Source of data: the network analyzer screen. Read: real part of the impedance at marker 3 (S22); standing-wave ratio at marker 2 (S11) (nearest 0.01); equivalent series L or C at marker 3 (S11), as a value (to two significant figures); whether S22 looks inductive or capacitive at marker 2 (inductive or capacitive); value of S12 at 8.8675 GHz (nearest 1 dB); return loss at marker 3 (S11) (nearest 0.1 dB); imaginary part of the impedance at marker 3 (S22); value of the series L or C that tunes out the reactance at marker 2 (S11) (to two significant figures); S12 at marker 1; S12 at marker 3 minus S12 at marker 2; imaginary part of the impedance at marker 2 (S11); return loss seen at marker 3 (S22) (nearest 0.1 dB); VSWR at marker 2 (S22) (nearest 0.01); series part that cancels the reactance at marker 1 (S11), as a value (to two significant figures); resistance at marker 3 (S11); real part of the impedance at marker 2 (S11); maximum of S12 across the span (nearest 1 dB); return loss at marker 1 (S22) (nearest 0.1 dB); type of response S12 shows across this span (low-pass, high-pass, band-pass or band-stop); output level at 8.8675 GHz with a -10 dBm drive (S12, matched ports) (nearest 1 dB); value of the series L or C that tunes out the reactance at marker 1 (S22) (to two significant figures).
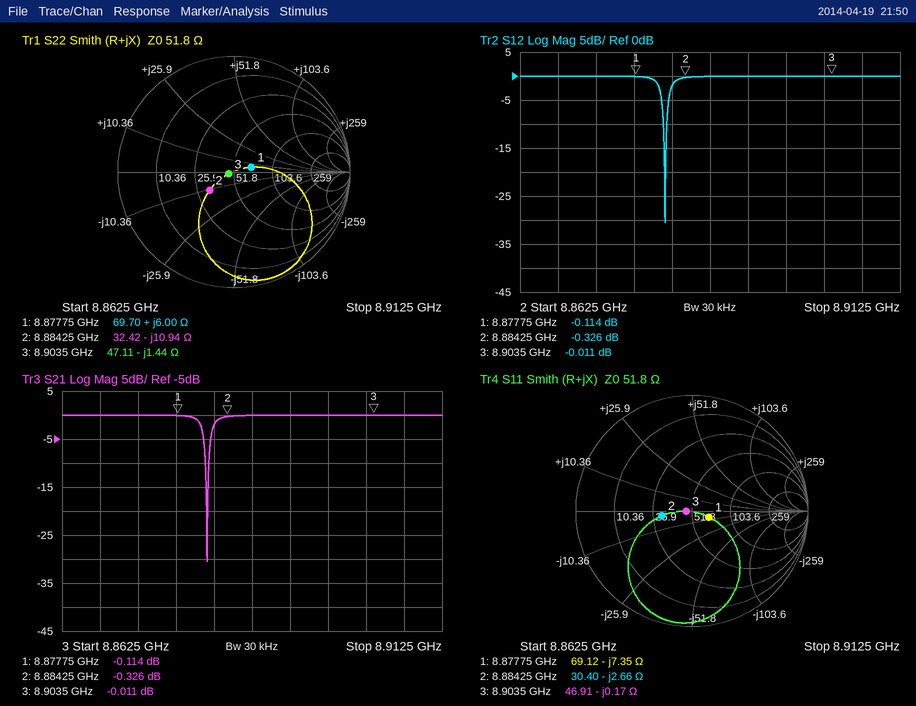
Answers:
47.11 Ω
1.71
110 pF
capacitive
0 dB
26.1 dB
-1.44 Ω
48 pH
-0.114 dB
0.315 dB
-2.66 Ω
26.1 dB
1.71
130 pH
46.91 Ω
30.40 Ω
0 dB
16.2 dB
band-stop
-10 dBm
3.0 pF
